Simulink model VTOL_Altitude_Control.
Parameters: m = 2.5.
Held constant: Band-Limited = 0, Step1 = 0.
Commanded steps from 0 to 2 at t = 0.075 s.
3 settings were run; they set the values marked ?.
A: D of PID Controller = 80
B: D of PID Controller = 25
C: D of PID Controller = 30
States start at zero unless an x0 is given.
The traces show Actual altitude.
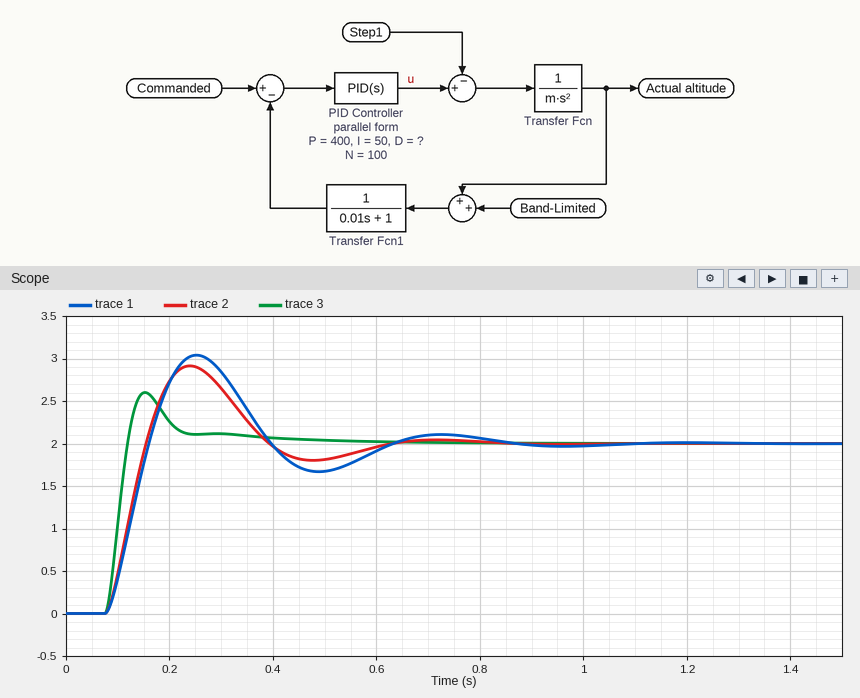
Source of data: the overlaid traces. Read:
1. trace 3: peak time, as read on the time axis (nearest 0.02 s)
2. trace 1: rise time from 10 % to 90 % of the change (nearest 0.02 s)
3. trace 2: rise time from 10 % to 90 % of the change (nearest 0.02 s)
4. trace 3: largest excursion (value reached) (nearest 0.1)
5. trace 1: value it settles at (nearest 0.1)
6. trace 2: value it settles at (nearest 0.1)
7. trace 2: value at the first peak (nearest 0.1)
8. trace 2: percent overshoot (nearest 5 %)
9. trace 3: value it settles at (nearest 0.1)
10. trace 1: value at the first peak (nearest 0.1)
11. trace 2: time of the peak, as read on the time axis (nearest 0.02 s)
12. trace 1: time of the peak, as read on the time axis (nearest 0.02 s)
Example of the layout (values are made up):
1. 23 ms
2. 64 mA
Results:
1. 0.16 s
2. 0.06 s
3. 0.06 s
4. 2.6
5. 2.0
6. 2.0
7. 2.9
8. 45 %
9. 2.0
10. 3.0
11. 0.24 s
12. 0.26 s
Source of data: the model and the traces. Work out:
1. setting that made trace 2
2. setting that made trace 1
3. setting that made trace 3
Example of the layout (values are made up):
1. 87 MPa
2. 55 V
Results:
1. C
2. B
3. A
